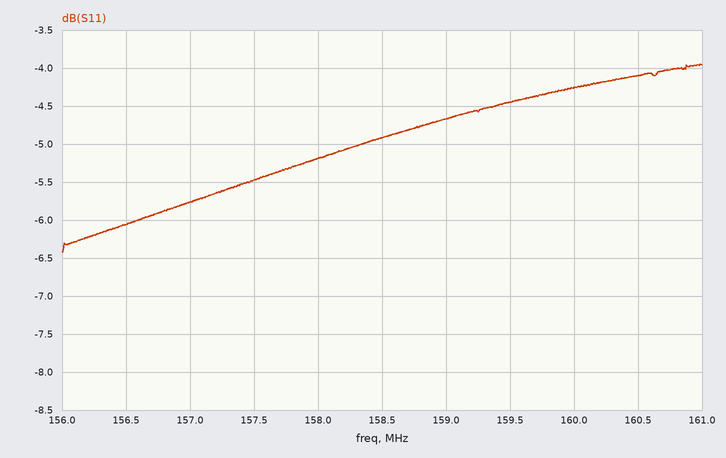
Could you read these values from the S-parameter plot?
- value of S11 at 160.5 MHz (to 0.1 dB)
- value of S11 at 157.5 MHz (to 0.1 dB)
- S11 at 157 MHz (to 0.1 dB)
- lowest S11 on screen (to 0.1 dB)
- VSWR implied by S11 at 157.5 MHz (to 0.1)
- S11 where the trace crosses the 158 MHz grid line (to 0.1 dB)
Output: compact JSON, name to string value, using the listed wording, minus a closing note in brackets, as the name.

{"value of S11 at 160.5 MHz": "-4.1 dB", "value of S11 at 157.5 MHz": "-5.5 dB", "S11 at 157 MHz": "-5.8 dB", "lowest S11 on screen": "-6.4 dB", "VSWR implied by S11 at 157.5 MHz": "3.3", "S11 where the trace crosses the 158 MHz grid line": "-5.2 dB"}
